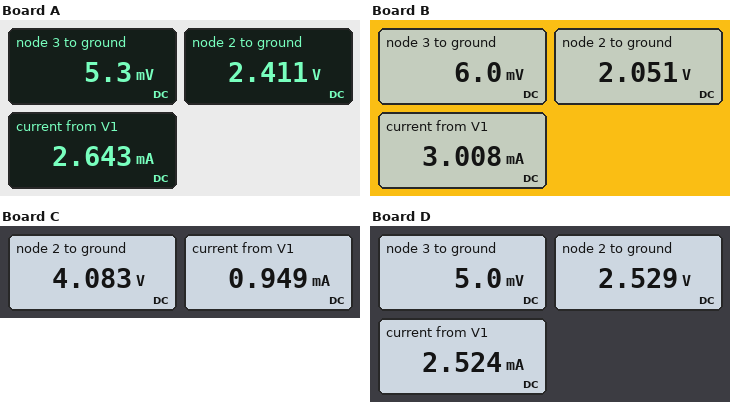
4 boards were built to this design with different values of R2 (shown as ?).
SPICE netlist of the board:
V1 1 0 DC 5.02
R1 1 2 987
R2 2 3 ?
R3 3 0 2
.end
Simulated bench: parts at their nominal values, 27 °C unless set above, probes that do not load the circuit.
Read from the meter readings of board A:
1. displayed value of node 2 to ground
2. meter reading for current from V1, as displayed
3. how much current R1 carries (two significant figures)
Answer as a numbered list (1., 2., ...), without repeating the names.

1. 2.411 V
2. 2.643 mA
3. 2.6 mA
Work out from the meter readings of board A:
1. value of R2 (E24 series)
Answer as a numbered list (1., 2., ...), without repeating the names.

1. 910 Ω
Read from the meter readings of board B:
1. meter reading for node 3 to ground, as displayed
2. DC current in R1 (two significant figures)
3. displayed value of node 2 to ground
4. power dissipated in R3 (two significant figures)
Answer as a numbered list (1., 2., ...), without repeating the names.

1. 6.0 mV
2. 3.0 mA
3. 2.051 V
4. 18 µW
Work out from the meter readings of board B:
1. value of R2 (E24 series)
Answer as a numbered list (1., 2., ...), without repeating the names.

1. 680 Ω
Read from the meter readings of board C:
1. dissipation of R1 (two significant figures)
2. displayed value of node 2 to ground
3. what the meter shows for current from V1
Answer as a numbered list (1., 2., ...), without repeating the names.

1. 890 µW
2. 4.083 V
3. 0.949 mA
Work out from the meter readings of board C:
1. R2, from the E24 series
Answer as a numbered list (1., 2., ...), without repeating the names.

1. 4.3 kΩ
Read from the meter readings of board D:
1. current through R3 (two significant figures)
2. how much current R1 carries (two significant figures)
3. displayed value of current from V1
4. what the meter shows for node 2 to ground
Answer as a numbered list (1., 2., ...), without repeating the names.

1. 2.5 mA
2. 2.5 mA
3. 2.524 mA
4. 2.529 V
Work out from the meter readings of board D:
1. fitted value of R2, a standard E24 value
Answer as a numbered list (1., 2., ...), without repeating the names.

1. 1 kΩ
